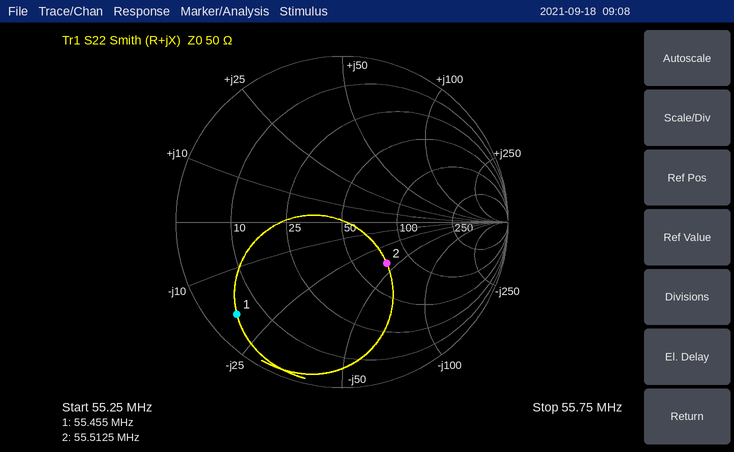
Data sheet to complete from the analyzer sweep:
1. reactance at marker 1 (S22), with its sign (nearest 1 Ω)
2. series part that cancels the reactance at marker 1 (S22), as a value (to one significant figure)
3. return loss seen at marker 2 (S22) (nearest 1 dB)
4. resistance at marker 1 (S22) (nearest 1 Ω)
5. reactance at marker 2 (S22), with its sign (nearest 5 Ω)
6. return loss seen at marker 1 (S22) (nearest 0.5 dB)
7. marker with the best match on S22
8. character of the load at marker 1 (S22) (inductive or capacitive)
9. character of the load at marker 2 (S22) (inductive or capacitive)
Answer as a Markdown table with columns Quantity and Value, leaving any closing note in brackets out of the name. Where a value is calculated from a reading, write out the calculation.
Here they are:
| Quantity | Value |
|---|---|
| reactance at marker 1 (S22), with its sign | -19 Ω |
| series part that cancels the reactance at marker 1 (S22), as a value | L = 19 Ω/(2π × 55.455 MHz) ≈ 54.5 nH, so 50 nH to one significant figure |
| return loss seen at marker 2 (S22) | 9 dB |
| resistance at marker 1 (S22) | 5 Ω |
| reactance at marker 2 (S22), with its sign | -40 Ω |
| return loss seen at marker 1 (S22) | 1.5 dB |
| marker with the best match on S22 | marker 2 |
| character of the load at marker 1 (S22) | capacitive |
| character of the load at marker 2 (S22) | capacitive |
